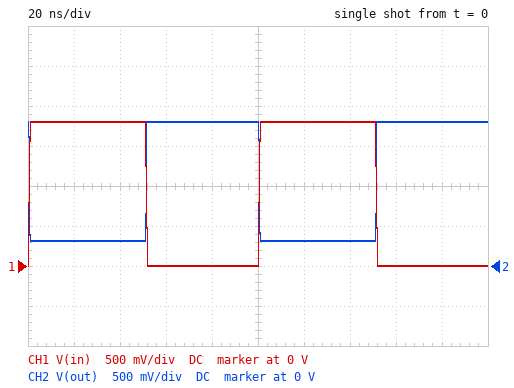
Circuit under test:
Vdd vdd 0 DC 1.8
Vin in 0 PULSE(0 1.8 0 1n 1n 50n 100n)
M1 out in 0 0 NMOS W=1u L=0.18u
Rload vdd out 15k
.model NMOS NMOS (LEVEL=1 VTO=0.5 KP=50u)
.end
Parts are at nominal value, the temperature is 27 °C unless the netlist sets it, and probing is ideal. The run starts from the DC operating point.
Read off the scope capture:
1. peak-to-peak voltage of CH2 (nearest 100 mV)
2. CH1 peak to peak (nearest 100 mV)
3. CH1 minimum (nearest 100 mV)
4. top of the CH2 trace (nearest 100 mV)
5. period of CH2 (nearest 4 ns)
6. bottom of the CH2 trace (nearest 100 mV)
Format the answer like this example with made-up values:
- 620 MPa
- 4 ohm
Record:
- 1.5 V
- 1.8 V
- 0 V
- 1.8 V
- 100 ns
- 300 mV
